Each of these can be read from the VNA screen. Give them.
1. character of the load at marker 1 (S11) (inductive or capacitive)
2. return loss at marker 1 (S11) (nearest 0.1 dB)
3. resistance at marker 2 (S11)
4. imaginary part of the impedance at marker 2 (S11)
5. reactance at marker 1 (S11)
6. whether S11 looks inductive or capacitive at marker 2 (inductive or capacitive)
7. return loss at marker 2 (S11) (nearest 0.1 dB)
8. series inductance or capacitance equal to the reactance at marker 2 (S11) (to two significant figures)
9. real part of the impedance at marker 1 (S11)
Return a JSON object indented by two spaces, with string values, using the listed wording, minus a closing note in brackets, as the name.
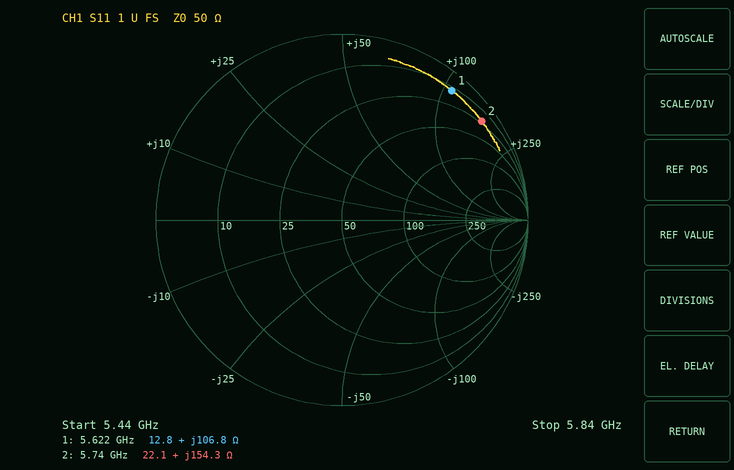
{
  "character of the load at marker 1 (S11)": "inductive",
  "return loss at marker 1 (S11)": "0.8 dB",
  "resistance at marker 2": "22.1 Ω",
  "imaginary part of the impedance at marker 2": "+154.3 Ω",
  "reactance at marker 1": "+106.8 Ω",
  "whether S11 looks inductive or capacitive at marker 2": "inductive",
  "return loss at marker 2 (S11)": "0.7 dB",
  "series inductance or capacitance equal to the reactance at marker 2 (S11)": "4.3 nH",
  "real part of the impedance at marker 1": "12.8 Ω"
}
